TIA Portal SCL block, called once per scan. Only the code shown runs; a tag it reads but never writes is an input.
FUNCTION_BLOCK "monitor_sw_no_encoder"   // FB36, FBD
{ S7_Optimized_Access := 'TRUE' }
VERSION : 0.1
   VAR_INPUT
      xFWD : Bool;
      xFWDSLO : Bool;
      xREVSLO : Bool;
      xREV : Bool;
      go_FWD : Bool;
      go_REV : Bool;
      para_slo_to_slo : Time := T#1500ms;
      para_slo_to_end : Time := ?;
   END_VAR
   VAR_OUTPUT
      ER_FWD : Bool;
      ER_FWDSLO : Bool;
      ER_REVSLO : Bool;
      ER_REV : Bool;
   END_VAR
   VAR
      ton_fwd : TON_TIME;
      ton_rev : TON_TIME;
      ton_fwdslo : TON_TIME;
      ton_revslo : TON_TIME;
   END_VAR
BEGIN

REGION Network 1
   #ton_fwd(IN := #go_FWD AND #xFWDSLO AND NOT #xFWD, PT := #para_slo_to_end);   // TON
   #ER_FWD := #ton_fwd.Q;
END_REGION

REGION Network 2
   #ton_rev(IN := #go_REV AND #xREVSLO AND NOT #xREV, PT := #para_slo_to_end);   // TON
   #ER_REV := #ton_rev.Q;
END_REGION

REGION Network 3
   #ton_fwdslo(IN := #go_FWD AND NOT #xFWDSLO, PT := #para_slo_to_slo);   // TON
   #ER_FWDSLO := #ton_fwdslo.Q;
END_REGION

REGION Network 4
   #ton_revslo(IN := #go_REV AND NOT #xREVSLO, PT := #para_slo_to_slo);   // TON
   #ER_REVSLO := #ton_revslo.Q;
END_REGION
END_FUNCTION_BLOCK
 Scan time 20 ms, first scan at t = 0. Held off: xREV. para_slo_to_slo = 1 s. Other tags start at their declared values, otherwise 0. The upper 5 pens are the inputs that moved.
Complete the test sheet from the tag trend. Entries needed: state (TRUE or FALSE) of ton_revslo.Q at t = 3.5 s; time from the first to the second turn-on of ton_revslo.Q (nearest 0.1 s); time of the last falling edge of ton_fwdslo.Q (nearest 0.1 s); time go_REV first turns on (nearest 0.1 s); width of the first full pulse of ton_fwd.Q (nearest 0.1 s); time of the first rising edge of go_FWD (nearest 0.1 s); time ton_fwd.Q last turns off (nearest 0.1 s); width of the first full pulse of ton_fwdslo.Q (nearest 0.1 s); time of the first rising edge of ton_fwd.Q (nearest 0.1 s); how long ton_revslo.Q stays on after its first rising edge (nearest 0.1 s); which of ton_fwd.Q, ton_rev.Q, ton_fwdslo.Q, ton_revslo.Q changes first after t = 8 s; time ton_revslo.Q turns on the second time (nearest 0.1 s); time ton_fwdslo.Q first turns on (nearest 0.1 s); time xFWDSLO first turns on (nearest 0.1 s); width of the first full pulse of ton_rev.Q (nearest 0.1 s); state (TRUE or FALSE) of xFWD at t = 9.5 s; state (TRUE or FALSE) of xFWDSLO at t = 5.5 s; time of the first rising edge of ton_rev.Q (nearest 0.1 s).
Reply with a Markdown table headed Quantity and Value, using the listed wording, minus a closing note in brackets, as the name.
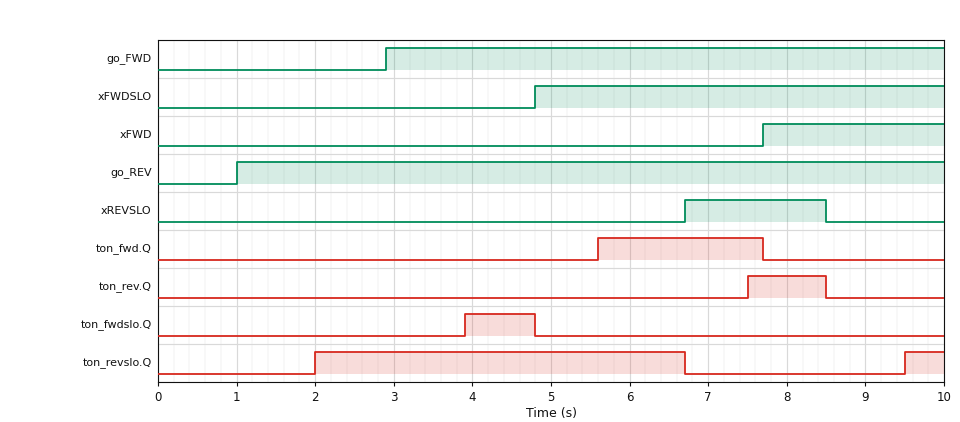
| Quantity | Value |
|---|---|
| state (TRUE or FALSE) of ton_revslo.Q at t = 3.5 s | TRUE |
| time from the first to the second turn-on of ton_revslo.Q | 7.5 s |
| time of the last falling edge of ton_fwdslo.Q | 4.8 s |
| time go_REV first turns on | 1.0 s |
| width of the first full pulse of ton_fwd.Q | 2.1 s |
| time of the first rising edge of go_FWD | 2.9 s |
| time ton_fwd.Q last turns off | 7.7 s |
| width of the first full pulse of ton_fwdslo.Q | 0.9 s |
| time of the first rising edge of ton_fwd.Q | 5.6 s |
| how long ton_revslo.Q stays on after its first rising edge | 4.7 s |
| which of ton_fwd.Q, ton_rev.Q, ton_fwdslo.Q, ton_revslo.Q changes first after t = 8 s | ton_rev.Q |
| time ton_revslo.Q turns on the second time | 9.5 s |
| time ton_fwdslo.Q first turns on | 3.9 s |
| time xFWDSLO first turns on | 4.8 s |
| width of the first full pulse of ton_rev.Q | 1.0 s |
| state (TRUE or FALSE) of xFWD at t = 9.5 s | TRUE |
| state (TRUE or FALSE) of xFWDSLO at t = 5.5 s | TRUE |
| time of the first rising edge of ton_rev.Q | 7.5 s |
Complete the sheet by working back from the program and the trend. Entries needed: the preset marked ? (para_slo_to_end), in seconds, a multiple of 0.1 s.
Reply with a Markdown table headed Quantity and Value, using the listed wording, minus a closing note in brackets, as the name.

| Quantity | Value |
|---|---|
| the preset marked ? (para_slo_to_end), in seconds, a multiple of 0.1 s | 0.8 s |
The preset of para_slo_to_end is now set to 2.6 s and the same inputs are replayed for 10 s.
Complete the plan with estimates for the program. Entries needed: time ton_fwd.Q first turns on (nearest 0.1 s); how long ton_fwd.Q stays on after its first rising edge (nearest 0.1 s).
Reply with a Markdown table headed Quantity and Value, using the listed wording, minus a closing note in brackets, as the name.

| Quantity | Value |
|---|---|
| time ton_fwd.Q first turns on | 7.4 s |
| how long ton_fwd.Q stays on after its first rising edge | 0.3 s |
